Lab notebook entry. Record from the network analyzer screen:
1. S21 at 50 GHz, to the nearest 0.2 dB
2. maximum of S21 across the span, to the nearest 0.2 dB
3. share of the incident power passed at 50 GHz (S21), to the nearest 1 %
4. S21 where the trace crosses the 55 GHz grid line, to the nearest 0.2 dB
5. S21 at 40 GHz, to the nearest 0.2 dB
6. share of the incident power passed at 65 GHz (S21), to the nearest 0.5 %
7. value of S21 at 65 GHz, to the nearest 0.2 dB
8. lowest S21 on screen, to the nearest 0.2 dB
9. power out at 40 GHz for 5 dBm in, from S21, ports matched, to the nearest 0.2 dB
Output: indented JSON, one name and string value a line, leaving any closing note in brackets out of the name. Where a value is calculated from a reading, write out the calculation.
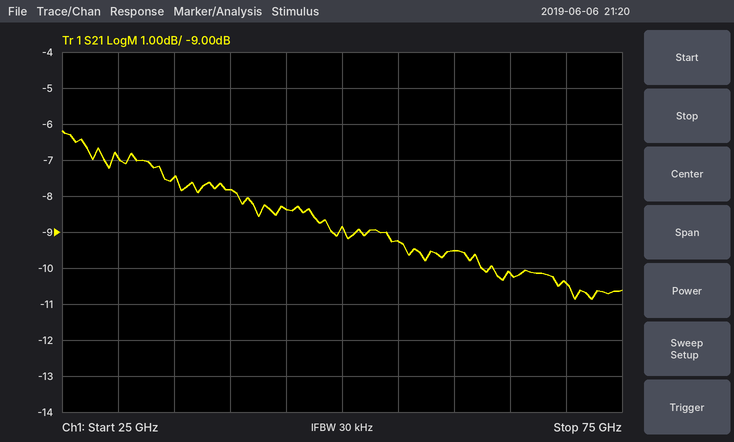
{
  "S21 at 50 GHz, to the nearest 0.2 dB": "-8.8 dB",
  "maximum of S21 across the span, to the nearest 0.2 dB": "-6.2 dB",
  "share of the incident power passed at 50 GHz (S21), to the nearest 1 %": "10^(-8.8/10) ≈ 13 %",
  "S21 where the trace crosses the 55 GHz grid line, to the nearest 0.2 dB": "-9.2 dB",
  "S21 at 40 GHz, to the nearest 0.2 dB": "-7.8 dB",
  "share of the incident power passed at 65 GHz (S21), to the nearest 0.5 %": "10^(-10.2/10) ≈ 9.5 %",
  "value of S21 at 65 GHz, to the nearest 0.2 dB": "-10.2 dB",
  "lowest S21 on screen, to the nearest 0.2 dB": "-10.8 dB",
  "power out at 40 GHz for 5 dBm in, from S21, ports matched, to the nearest 0.2 dB": "5 dBm + (-7.8 dB) = -2.8 dBm"
}
